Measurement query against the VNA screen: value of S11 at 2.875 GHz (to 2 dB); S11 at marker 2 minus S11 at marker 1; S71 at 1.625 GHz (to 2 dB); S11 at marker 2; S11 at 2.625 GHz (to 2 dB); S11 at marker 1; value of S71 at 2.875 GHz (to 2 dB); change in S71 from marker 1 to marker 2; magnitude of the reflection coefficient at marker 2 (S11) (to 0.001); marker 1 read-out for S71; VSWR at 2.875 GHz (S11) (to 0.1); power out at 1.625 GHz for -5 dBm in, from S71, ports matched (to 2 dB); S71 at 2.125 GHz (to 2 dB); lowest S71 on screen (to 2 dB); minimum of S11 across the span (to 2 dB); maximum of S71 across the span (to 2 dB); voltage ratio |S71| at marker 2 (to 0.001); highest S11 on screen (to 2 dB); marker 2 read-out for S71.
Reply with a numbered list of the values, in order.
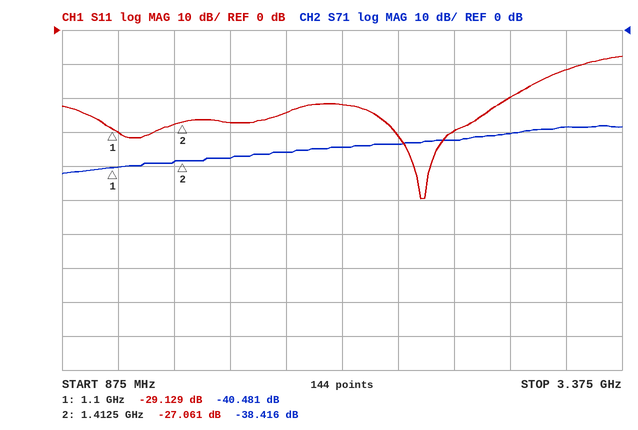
1. -20 dB
2. 2.068 dB
3. -38 dB
4. -27.061 dB
5. -30 dB
6. -29.129 dB
7. -30 dB
8. 2.065 dB
9. 0.044
10. -40.481 dB
11. 1.2
12. -42 dBm
13. -34 dB
14. -42 dB
15. -50 dB
16. -28 dB
17. 0.012
18. -8 dB
19. -38.416 dB
